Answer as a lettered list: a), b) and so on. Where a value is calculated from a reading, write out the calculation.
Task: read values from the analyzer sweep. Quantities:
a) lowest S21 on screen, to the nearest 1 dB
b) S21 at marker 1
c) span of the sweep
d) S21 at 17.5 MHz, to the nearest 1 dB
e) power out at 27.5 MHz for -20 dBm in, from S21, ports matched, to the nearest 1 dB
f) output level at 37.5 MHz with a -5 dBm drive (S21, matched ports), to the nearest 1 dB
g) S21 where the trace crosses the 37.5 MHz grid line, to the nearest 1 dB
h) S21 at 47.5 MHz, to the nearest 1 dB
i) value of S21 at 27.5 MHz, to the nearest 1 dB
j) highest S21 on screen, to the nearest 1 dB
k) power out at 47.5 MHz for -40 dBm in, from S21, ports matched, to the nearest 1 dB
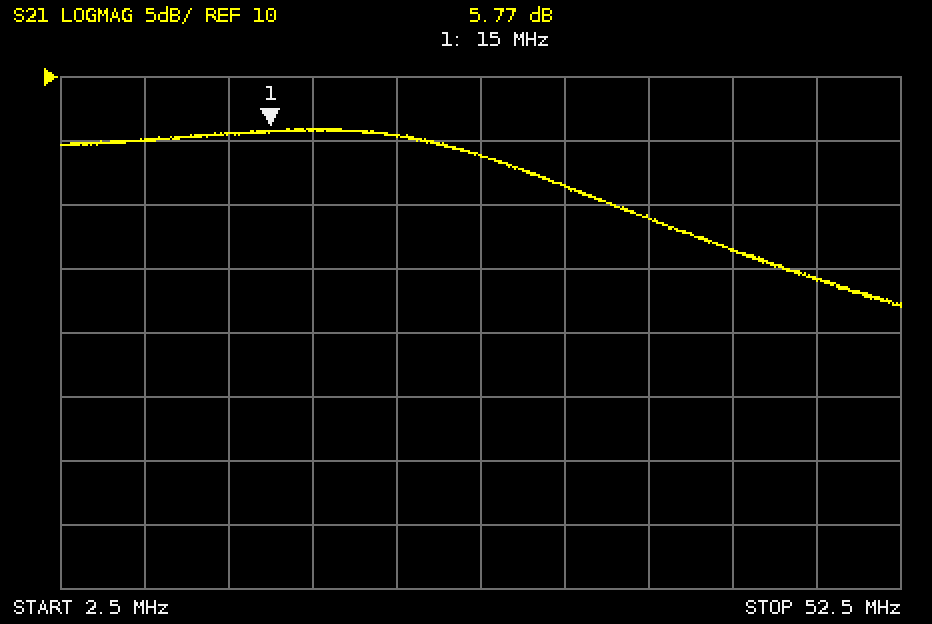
a) -8 dB
b) 5.77 dB
c) 50 MHz
d) 6 dB
e) -20 dBm + (4 dB) = -16 dBm
f) -5 dBm + (-1 dB) = -6 dBm
g) -1 dB
h) -6 dB
i) 4 dB
j) 6 dB
k) -40 dBm + (-6 dB) = -46 dBm
